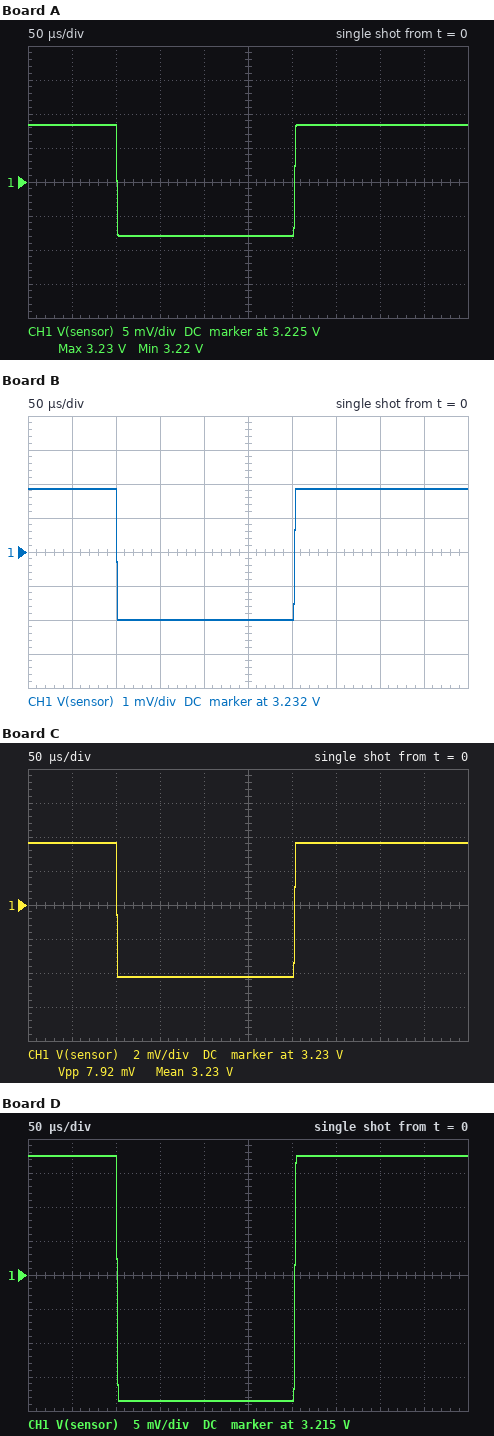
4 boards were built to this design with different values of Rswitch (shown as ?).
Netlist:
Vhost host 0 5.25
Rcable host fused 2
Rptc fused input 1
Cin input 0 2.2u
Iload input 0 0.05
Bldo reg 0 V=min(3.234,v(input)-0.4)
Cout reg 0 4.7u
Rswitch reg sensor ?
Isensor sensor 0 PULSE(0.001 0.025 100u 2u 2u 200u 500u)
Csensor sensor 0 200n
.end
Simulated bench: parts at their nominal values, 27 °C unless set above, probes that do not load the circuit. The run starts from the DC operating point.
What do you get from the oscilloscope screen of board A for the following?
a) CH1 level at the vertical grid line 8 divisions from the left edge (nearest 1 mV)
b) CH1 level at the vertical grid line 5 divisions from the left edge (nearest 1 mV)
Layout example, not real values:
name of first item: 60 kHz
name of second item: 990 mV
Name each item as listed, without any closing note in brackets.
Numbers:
CH1 level at the vertical grid line 8 divisions from the left edge: 3.233 V
CH1 level at the vertical grid line 5 divisions from the left edge: 3.217 V
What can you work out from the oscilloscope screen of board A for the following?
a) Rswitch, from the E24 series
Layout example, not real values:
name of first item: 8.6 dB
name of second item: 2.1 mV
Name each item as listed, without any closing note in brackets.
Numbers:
Rswitch, from the E24 series: 0.68 Ω
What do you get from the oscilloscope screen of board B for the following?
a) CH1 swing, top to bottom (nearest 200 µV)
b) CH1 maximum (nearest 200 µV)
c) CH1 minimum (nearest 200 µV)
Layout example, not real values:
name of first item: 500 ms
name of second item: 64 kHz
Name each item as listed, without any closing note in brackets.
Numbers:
CH1 swing, top to bottom: 3.8 mV
CH1 maximum: 3.2338 V
CH1 minimum: 3.2300 V
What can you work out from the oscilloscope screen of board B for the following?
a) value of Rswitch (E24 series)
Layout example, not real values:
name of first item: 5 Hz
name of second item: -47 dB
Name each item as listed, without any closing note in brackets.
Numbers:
value of Rswitch: 0.16 Ω
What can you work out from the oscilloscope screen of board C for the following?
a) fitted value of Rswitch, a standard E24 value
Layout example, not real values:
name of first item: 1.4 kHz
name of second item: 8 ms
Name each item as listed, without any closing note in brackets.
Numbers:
fitted value of Rswitch, a standard E24 value: 0.33 Ω
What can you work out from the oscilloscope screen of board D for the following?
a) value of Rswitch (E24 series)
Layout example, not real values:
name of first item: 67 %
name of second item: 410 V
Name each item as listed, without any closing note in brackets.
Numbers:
value of Rswitch: 1.5 Ω
